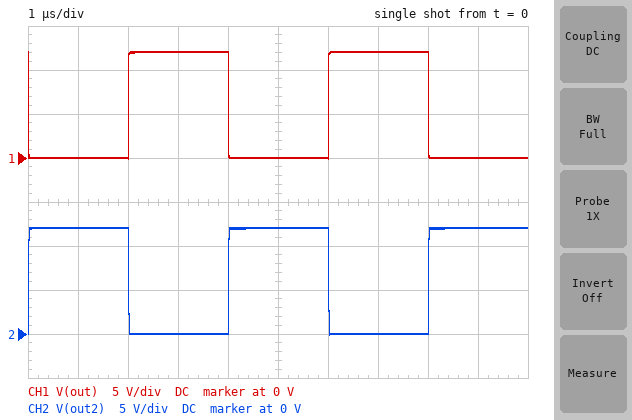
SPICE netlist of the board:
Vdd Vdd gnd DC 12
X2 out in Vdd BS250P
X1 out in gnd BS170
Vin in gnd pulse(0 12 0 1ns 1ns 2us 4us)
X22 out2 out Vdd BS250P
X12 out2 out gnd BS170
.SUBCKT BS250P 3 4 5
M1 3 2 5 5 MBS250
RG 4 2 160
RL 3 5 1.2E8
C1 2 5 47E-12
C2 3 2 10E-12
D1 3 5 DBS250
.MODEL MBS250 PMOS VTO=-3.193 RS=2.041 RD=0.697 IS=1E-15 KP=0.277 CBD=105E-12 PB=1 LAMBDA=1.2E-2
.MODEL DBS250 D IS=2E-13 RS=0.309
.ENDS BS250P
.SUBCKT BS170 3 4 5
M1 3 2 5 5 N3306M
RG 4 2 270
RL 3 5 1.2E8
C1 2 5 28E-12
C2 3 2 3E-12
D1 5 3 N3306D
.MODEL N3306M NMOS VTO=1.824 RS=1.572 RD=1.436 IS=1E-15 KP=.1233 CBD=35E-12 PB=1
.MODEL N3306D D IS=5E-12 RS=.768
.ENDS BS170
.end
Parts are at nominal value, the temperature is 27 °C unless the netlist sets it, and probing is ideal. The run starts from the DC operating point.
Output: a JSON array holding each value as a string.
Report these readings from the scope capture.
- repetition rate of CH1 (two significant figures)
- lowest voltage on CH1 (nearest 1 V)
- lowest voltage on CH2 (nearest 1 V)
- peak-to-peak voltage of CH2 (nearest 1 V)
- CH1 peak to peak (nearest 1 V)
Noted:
["250 kHz", "0 V", "0 V", "12 V", "12 V"]
